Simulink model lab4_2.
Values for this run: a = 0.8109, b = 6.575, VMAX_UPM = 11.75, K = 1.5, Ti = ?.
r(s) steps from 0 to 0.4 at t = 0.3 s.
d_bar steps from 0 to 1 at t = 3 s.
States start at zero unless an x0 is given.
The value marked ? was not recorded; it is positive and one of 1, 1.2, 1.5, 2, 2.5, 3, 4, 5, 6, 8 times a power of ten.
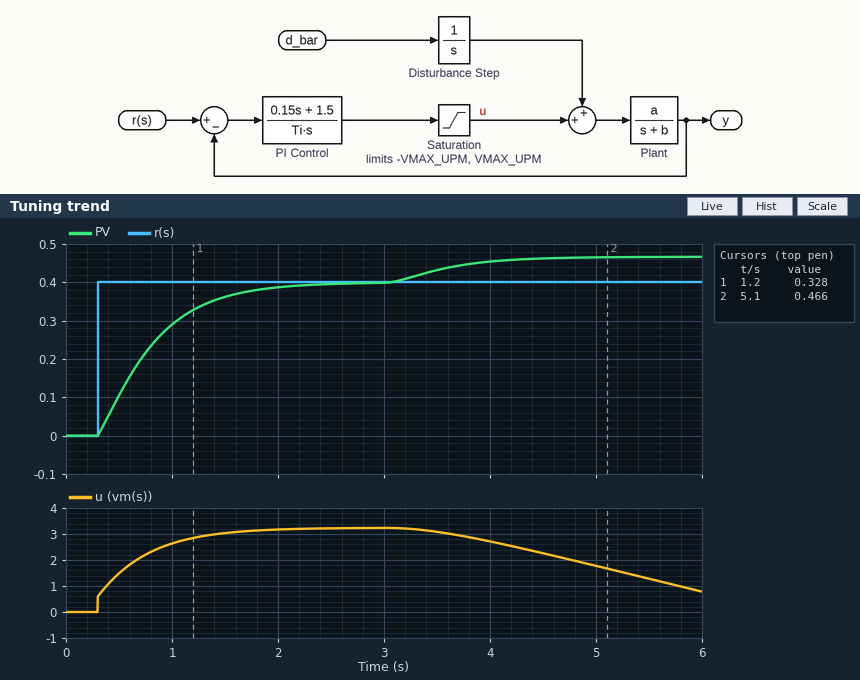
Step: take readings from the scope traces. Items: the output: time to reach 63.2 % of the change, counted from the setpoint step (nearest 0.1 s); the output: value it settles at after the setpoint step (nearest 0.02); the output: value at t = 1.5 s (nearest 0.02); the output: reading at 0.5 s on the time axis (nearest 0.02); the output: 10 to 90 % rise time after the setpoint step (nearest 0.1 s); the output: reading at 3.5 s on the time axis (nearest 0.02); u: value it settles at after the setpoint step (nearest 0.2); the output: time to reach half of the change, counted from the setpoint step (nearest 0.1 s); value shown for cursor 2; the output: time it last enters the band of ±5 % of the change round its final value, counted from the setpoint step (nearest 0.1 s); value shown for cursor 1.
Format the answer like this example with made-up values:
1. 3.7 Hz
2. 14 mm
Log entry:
1. 0.6 s
2. 0.40
3. 0.36
4. 0.10
5. 1.1 s
6. 0.44
7. 3.2
8. 0.4 s
9. 0.466
10. 1.5 s
11. 0.328
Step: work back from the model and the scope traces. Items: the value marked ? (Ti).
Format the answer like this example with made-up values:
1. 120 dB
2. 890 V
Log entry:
1. 0.1
